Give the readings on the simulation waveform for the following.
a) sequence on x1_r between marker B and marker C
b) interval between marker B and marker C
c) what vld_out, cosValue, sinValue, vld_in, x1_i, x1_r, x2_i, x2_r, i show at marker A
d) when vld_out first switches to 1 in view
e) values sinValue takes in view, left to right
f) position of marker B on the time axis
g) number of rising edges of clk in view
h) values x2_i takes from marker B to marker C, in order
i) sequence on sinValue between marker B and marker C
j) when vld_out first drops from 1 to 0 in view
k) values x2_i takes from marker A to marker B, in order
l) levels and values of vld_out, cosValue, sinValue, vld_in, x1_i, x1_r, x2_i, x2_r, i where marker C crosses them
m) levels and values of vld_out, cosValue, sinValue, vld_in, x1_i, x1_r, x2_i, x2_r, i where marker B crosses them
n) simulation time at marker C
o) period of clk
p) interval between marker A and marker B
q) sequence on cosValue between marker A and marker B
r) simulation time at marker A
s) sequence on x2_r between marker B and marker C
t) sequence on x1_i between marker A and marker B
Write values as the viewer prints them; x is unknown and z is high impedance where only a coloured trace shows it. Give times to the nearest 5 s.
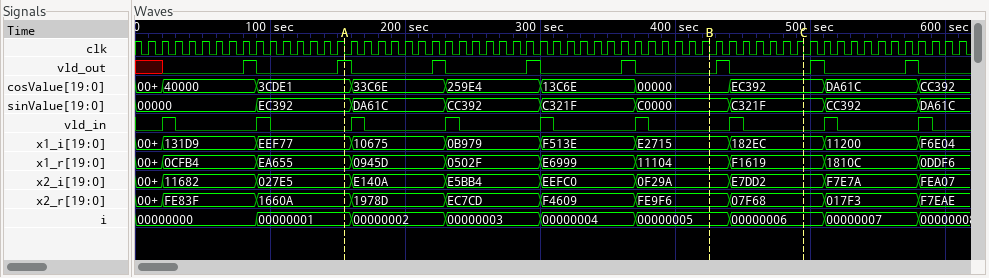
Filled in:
11104, F1619
70 s
vld_out=1, cosValue=3CDE1, sinValue=EC392, vld_in=0, x1_i=EEF77, x1_r=EA655, x2_i=027E5, x2_r=1660A, i=00000001
80 s
00000, EC392, DA61C, CC392, C321F, C0000, C321F, CC392, DA61C
425 s
61
0F29A, E7DD2
C0000, C321F
90 s
027E5, E140A, E5BB4, EEFC0, 0F29A
vld_out=0, cosValue=EC392, sinValue=C321F, vld_in=0, x1_i=182EC, x1_r=F1619, x2_i=E7DD2, x2_r=07F68, i=00000006
vld_out=0, cosValue=00000, sinValue=C0000, vld_in=0, x1_i=E2715, x1_r=11104, x2_i=0F29A, x2_r=FE9F6, i=00000005
495 s
10 s
270 s
3CDE1, 33C6E, 259E4, 13C6E, 00000
155 s
FE9F6, 07F68
EEF77, 10675, 0B979, F513E, E2715
